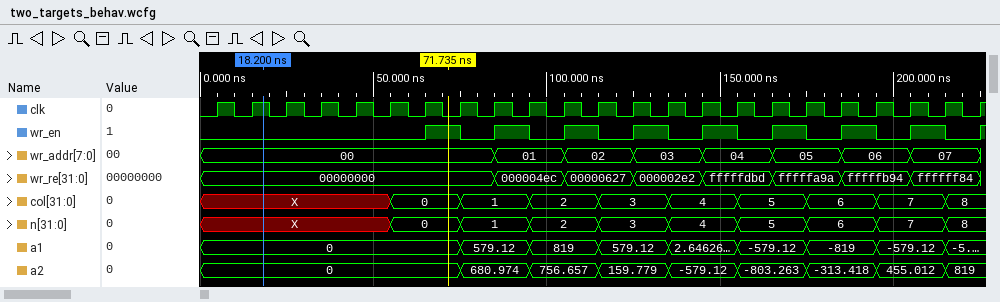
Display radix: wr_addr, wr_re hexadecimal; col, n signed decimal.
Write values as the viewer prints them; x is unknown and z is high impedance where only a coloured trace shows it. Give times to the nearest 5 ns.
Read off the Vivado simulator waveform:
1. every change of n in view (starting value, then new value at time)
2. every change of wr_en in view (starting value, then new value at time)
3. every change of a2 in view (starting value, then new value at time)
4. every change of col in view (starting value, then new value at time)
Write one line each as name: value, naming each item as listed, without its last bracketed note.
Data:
every change of n in view: X, 0 at 55 ns, 1 at 75 ns, 2 at 95 ns, 3 at 115 ns, 4 at 135 ns, 5 at 155 ns, 6 at 175 ns, 7 at 195 ns, 8 at 215 ns
every change of wr_en in view: 0, 1 at 65 ns, 0 at 75 ns, 1 at 85 ns, 0 at 95 ns, 1 at 105 ns, 0 at 115 ns, 1 at 125 ns, 0 at 135 ns, 1 at 145 ns, 0 at 155 ns, 1 at 165 ns, 0 at 175 ns, 1 at 185 ns, 0 at 195 ns, 1 at 205 ns, 0 at 215 ns, 1 at 225 ns
every change of a2 in view: 0, 680.974 at 75 ns, 756.657 at 95 ns, 159.779 at 115 ns, -579.12 at 135 ns, -803.263 at 155 ns, -313.418 at 175 ns, 455.012 at 195 ns, 819 at 215 ns
every change of col in view: X, 0 at 55 ns, 1 at 75 ns, 2 at 95 ns, 3 at 115 ns, 4 at 135 ns, 5 at 155 ns, 6 at 175 ns, 7 at 195 ns, 8 at 215 ns
